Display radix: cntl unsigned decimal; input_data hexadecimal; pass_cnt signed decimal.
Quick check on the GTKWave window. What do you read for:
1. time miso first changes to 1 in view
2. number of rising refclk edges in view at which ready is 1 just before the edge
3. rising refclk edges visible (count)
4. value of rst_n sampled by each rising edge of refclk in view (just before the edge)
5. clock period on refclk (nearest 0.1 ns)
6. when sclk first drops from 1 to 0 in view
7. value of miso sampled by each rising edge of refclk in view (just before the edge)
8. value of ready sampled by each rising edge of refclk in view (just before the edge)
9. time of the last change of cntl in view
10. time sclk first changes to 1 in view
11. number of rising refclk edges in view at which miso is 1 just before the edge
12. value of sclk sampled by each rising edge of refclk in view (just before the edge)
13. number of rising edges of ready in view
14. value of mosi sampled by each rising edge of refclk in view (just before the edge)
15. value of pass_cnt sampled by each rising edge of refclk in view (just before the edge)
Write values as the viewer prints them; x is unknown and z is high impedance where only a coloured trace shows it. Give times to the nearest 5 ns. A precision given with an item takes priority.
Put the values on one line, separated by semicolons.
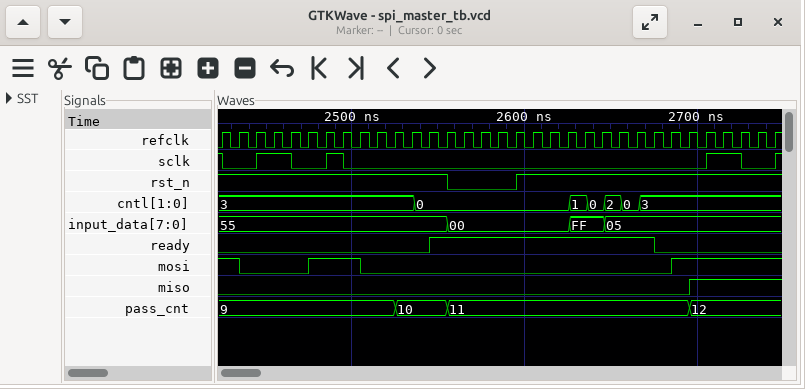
2695 ns; 13; 33; 1 1 1 1 1 1 1 1 1 1 1 1 1 1 0 0 0 0 1 1 1 1 1 1 1 1 1 1 1 1 1 1 1; 10 ns; 2425 ns; 0 0 0 0 0 0 0 0 0 0 0 0 0 0 0 0 0 0 0 0 0 0 0 0 0 0 0 0 1 1 1 1 1; 0 0 0 0 0 0 0 0 0 0 0 0 0 1 1 1 1 1 1 1 1 1 1 1 1 1 0 0 0 0 0 0 0; 2665 ns; 2445 ns; 5; 1 0 0 1 1 0 0 1 0 0 0 0 0 0 0 0 0 0 0 0 0 0 0 0 0 0 0 0 0 1 1 0 0; 1; 1 1 0 0 0 0 1 1 1 0 0 0 0 0 0 0 0 0 0 0 0 0 0 0 0 0 0 1 1 1 1 1 1; 9, 9, 9, 9, 9, 9, 9, 9, 9, 9, 9, 10, 10, 10, 11, 11, 11, 11, 11, 11, 11, 11, 11, 11, 11, 11, 11, 11, 12, 12, 12, 12, 12
